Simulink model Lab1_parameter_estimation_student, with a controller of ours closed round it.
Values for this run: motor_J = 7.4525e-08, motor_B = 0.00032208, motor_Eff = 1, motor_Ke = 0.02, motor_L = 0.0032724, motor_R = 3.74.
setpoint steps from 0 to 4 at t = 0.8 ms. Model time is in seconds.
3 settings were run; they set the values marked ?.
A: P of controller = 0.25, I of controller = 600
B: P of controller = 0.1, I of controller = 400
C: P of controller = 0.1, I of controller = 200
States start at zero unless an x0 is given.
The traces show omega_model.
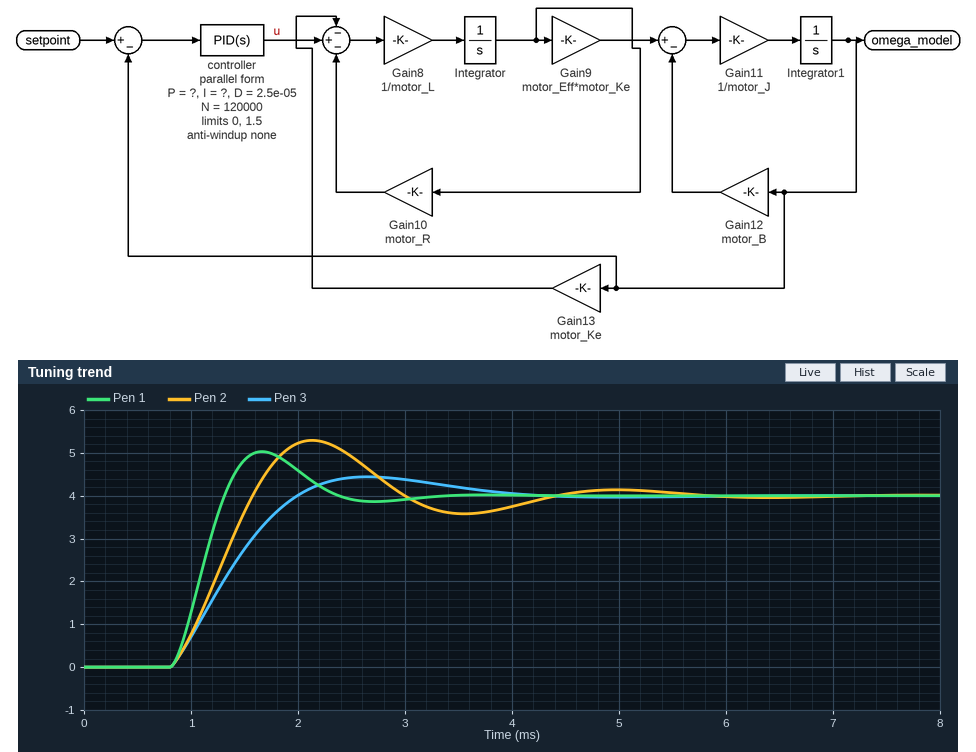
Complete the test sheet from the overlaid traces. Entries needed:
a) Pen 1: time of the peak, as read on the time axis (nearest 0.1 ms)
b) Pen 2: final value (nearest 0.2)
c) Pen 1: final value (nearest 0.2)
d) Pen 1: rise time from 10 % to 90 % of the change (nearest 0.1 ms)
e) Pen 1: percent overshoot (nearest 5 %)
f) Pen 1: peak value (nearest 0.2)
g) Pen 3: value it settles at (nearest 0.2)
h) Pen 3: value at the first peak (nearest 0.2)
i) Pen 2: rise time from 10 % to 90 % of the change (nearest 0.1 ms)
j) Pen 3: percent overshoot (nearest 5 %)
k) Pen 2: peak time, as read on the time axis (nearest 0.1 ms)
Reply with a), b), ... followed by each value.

a) 1.7 ms
b) 4.0
c) 4.0
d) 0.4 ms
e) 25 %
f) 5.0
g) 4.0
h) 4.4
i) 0.6 ms
j) 10 %
k) 2.1 ms
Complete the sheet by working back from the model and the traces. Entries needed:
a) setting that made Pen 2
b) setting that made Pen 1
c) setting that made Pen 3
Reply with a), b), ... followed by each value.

a) B
b) A
c) C
